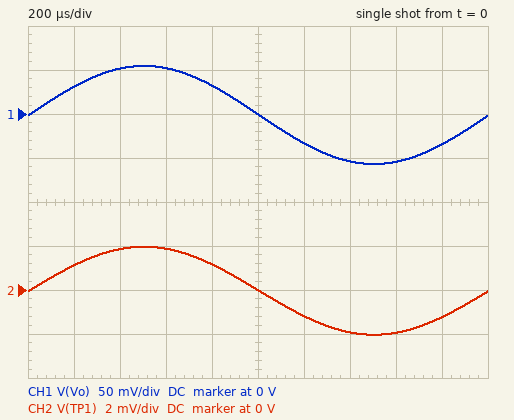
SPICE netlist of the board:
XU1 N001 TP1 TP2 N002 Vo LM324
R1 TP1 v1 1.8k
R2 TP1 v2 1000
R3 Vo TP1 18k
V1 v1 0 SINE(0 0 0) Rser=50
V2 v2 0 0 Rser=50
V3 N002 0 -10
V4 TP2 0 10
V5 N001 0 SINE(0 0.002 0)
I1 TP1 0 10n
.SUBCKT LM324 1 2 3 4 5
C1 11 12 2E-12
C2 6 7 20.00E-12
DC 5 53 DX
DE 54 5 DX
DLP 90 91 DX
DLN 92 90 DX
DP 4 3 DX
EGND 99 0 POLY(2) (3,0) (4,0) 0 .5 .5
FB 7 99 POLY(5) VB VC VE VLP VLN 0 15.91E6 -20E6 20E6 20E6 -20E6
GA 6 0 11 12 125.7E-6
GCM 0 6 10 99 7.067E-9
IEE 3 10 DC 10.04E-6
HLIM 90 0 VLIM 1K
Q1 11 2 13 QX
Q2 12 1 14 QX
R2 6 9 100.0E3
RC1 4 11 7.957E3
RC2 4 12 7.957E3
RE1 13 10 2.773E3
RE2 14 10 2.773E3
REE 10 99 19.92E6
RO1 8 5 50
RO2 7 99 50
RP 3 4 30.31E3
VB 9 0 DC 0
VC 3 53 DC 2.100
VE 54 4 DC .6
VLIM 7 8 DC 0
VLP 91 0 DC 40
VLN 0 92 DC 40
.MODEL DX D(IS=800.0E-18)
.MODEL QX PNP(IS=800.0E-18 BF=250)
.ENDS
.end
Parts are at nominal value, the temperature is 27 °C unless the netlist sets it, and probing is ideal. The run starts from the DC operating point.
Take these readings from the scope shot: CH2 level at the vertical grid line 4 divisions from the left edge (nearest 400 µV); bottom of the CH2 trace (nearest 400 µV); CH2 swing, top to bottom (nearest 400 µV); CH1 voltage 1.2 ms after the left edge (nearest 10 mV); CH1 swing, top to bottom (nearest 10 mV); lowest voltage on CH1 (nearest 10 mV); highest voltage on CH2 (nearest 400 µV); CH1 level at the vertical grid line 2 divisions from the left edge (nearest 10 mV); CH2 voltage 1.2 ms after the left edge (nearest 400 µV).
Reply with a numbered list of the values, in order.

1. 1.2 mV
2. -2.0 mV
3. 4.0 mV
4. -30 mV
5. 110 mV
6. -60 mV
7. 2.0 mV
8. 50 mV
9. -1.2 mV
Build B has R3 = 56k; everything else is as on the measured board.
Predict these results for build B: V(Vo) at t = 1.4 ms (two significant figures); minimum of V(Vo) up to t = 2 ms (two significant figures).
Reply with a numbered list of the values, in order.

1. -160 mV
2. -170 mV
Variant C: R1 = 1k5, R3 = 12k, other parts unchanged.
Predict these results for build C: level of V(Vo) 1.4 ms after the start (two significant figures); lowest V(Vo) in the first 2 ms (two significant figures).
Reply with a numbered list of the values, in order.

1. -39 mV
2. -41 mV
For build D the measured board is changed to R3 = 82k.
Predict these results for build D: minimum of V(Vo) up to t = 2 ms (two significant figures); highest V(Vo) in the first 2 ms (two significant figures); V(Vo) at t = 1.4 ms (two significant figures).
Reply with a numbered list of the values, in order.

1. -250 mV
2. 240 mV
3. -230 mV
